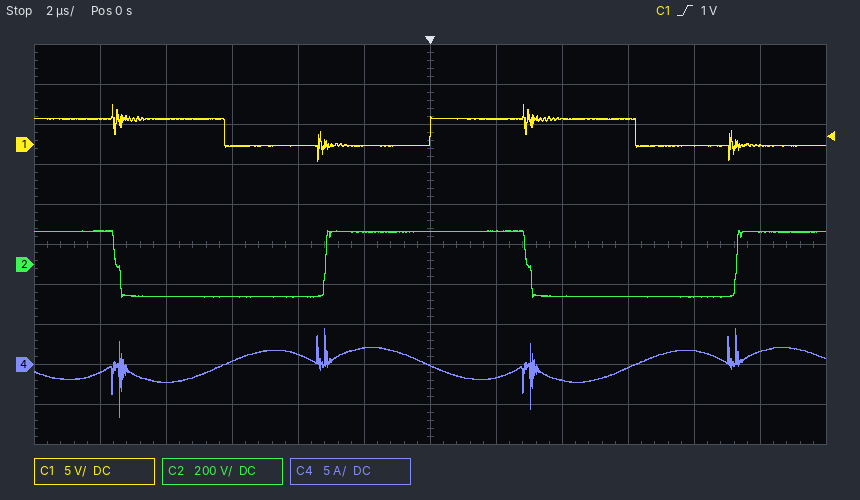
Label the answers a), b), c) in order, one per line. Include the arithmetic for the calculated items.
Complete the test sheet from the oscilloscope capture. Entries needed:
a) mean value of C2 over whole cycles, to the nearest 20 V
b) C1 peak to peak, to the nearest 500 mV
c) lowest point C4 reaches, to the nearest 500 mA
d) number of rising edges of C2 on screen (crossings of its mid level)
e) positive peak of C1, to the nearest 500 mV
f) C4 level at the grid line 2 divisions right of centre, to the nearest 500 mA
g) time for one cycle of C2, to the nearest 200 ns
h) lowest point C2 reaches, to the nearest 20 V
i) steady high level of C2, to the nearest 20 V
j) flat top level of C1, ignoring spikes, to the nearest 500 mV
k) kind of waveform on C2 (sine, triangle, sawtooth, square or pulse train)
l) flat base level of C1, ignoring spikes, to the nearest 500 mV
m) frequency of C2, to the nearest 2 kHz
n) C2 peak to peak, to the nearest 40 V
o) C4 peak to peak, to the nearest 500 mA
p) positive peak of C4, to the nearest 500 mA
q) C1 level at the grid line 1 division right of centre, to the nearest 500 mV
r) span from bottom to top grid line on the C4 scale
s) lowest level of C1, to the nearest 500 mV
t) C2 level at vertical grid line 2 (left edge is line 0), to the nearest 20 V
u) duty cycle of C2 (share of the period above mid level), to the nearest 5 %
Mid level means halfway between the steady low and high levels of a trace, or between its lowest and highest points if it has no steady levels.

a) -160 V + 0.5 × (160 V − (-160 V)) ≈ 0 V
b) 5.0 V − (-2.0 V) = 7.0 V
c) -6.5 A
d) 2
e) 5.0 V
f) -2.0 A
g) 12.4 µs
h) -160 V
i) 160 V
j) 3.0 V
k) square
l) 0.0 V
m) 1 / 12.4 µs ≈ 80.6 kHz, so 80 kHz to the nearest 2 kHz
n) 320 V
o) 4.5 A − (-6.5 A) = 11.0 A
p) 4.5 A
q) 3.0 V
r) 50 A
s) -2.0 V
t) -160 V
u) 50 %
